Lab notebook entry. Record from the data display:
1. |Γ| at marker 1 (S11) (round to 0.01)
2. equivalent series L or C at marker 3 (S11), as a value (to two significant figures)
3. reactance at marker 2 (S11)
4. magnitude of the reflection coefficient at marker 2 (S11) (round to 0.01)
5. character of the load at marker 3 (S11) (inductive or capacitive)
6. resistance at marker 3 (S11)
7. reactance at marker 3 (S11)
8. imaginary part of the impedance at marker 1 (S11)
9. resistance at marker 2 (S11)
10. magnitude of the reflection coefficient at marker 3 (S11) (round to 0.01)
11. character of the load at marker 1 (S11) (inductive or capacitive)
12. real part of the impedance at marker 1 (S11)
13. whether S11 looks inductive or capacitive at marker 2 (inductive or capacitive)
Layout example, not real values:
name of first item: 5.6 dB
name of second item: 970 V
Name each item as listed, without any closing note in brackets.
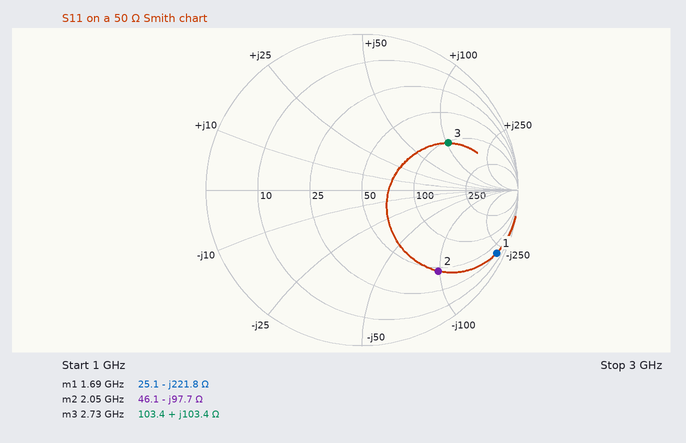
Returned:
|Γ| at marker 1 (S11): 0.95
equivalent series L or C at marker 3 (S11), as a value: 6.0 nH
reactance at marker 2: -97.7 Ω
magnitude of the reflection coefficient at marker 2 (S11): 0.71
character of the load at marker 3 (S11): inductive
resistance at marker 3: 103.4 Ω
reactance at marker 3: +103.4 Ω
imaginary part of the impedance at marker 1: -221.8 Ω
resistance at marker 2: 46.1 Ω
magnitude of the reflection coefficient at marker 3 (S11): 0.63
character of the load at marker 1 (S11): capacitive
real part of the impedance at marker 1: 25.1 Ω
whether S11 looks inductive or capacitive at marker 2: capacitive
